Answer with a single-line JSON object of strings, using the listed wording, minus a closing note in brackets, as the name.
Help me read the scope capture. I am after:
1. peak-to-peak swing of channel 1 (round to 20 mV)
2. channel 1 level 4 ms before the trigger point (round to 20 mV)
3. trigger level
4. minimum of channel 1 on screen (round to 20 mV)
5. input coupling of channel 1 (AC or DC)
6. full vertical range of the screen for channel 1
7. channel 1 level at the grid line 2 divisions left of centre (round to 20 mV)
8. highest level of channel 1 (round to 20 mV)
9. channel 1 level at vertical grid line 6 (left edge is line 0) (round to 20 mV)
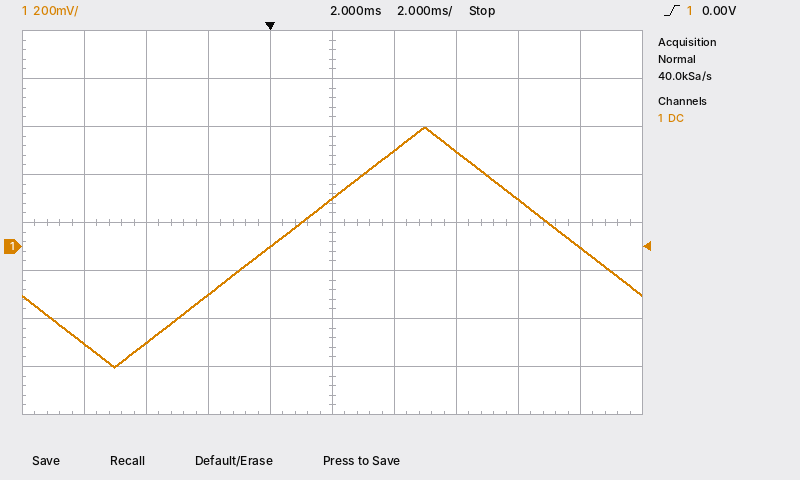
{"peak-to-peak swing of channel 1": "1.00 V", "channel 1 level 4 ms before the trigger point": "-400 mV", "trigger level": "0.00 V", "minimum of channel 1 on screen": "-500 mV", "input coupling of channel 1": "DC", "full vertical range of the screen for channel 1": "1.6 V", "channel 1 level at the grid line 2 divisions left of centre": "-200 mV", "highest level of channel 1": "500 mV", "channel 1 level at vertical grid line 6 (left edge is line 0)": "400 mV"}
